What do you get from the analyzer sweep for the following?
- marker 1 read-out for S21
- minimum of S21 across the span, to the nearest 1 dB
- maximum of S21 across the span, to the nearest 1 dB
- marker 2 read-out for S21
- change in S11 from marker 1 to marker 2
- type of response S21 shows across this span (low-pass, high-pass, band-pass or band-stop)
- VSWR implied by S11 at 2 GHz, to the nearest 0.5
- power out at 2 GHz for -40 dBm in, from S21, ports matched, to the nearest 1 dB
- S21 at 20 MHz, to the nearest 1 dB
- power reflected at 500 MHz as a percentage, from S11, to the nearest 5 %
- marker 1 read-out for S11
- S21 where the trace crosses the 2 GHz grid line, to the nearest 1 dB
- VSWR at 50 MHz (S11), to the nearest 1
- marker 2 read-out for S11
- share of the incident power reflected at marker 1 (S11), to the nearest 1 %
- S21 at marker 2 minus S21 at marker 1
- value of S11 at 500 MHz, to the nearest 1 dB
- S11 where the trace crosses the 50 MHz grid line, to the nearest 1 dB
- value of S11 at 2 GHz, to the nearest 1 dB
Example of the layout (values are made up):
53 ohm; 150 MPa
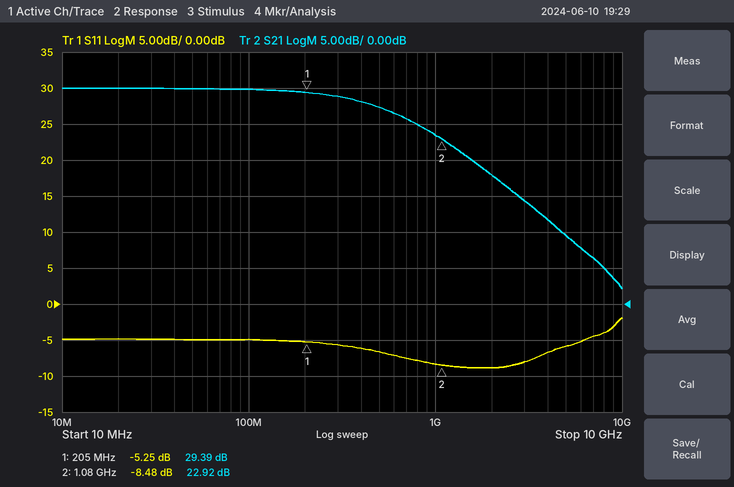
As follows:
29.39 dB; 2 dB; 30 dB; 22.92 dB; -3.23 dB; low-pass; 2.0; -22 dBm; 30 dB; 20 %; -5.25 dB; 18 dB; 4; -8.48 dB; 30 %; -6.47 dB; -7 dB; -5 dB; -9 dB
